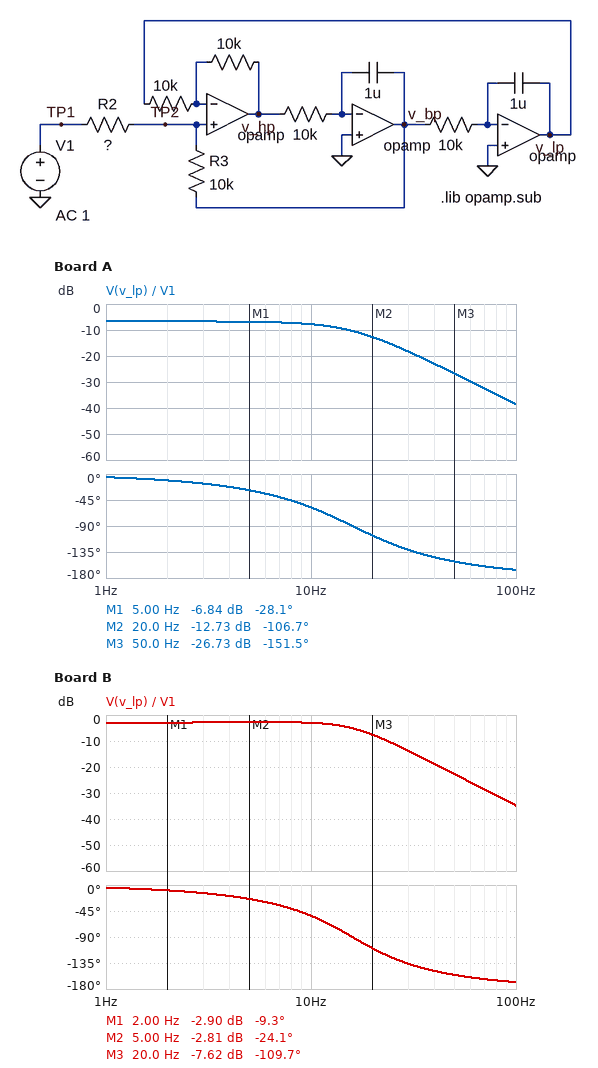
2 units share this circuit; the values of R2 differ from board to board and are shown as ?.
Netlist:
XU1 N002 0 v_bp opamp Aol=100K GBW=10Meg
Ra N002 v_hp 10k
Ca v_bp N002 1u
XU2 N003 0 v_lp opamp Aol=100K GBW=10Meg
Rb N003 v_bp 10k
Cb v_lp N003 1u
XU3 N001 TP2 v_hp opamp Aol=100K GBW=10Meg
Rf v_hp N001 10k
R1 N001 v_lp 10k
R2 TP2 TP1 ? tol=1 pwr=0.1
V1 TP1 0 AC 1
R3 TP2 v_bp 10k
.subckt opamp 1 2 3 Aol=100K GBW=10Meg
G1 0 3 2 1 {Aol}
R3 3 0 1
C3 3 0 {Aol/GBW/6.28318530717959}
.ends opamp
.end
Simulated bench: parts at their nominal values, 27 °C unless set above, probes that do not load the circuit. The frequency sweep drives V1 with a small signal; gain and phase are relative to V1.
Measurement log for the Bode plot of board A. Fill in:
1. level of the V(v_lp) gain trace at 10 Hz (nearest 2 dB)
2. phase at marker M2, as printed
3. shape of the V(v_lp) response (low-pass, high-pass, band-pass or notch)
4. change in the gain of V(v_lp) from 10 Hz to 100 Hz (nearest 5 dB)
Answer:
-8 dB
-106.7 deg
low-pass
-30 dB
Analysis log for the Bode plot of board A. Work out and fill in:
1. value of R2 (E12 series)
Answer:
33 kΩ
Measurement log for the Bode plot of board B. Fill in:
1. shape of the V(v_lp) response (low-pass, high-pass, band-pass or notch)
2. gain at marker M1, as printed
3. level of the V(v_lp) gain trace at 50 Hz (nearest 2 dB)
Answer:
low-pass
-2.90 dB
-22 dB
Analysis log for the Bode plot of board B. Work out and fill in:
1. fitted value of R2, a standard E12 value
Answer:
18 kΩ
